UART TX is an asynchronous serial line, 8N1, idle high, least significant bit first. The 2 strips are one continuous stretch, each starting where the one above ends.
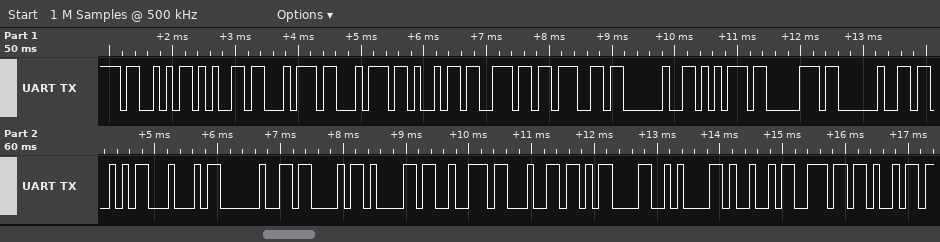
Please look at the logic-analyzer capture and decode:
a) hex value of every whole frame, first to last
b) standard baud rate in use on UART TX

53 65 74 74 69 6E 67 20 75 70 20 53 44 20 43 61 72 64 0D 0A 49 6E 69
9600 baud
